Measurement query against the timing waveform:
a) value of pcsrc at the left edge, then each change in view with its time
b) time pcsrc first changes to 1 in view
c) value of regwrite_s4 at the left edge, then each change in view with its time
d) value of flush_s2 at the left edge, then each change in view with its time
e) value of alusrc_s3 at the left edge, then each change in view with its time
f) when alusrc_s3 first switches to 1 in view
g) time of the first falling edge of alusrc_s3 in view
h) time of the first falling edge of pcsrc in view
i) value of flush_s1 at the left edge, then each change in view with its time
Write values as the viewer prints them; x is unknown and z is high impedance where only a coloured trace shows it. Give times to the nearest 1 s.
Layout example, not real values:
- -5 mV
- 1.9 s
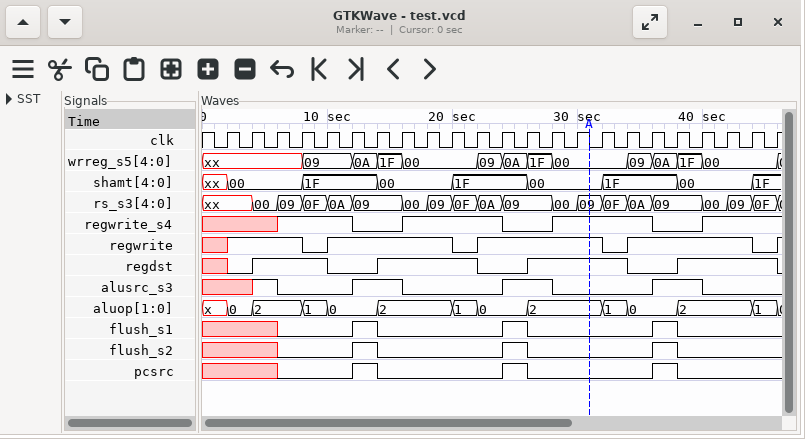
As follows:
- x, 0 at 6 s, 1 at 12 s, 0 at 14 s, 1 at 24 s, 0 at 26 s, 1 at 36 s, 0 at 38 s
- 12 s
- x, 1 at 6 s, 0 at 12 s, 1 at 16 s, 0 at 24 s, 1 at 28 s, 0 at 36 s, 1 at 40 s
- x, 0 at 6 s, 1 at 12 s, 0 at 14 s, 1 at 24 s, 0 at 26 s, 1 at 36 s, 0 at 38 s
- x, 1 at 4 s, 0 at 6 s, 1 at 12 s, 0 at 16 s, 1 at 24 s, 0 at 28 s, 1 at 36 s, 0 at 40 s
- 4 s
- 6 s
- 14 s
- x, 0 at 6 s, 1 at 12 s, 0 at 14 s, 1 at 24 s, 0 at 26 s, 1 at 36 s, 0 at 38 s
